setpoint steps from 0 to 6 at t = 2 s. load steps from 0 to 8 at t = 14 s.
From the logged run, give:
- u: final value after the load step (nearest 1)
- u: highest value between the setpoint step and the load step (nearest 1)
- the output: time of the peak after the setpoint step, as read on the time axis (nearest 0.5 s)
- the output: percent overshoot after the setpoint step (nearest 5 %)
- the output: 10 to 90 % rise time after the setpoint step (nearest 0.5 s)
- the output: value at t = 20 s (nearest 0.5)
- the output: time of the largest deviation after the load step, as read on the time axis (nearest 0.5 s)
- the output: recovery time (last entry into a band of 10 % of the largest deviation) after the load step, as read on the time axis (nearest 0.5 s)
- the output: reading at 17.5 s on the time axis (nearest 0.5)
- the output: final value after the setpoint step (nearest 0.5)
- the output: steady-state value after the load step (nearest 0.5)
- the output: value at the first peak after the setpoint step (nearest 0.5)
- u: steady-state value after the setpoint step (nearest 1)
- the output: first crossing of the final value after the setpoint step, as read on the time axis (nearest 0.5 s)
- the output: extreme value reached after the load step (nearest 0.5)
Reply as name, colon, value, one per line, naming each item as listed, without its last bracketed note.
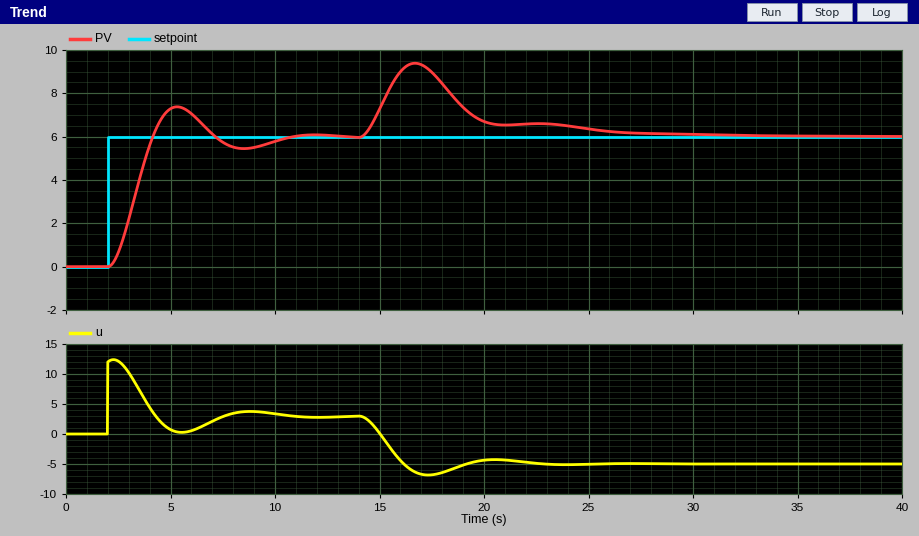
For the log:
u: final value after the load step: -5
u: highest value between the setpoint step and the load step: 12
the output: time of the peak after the setpoint step, as read on the time axis: 5.5 s
the output: percent overshoot after the setpoint step: 25 %
the output: 10 to 90 % rise time after the setpoint step: 1.5 s
the output: value at t = 20 s: 6.5
the output: time of the largest deviation after the load step, as read on the time axis: 16.5 s
the output: recovery time (last entry into a band of 10 % of the largest deviation) after the load step, as read on the time axis: 25.0 s
the output: reading at 17.5 s on the time axis: 9.0
the output: final value after the setpoint step: 6.0
the output: steady-state value after the load step: 6.0
the output: value at the first peak after the setpoint step: 7.5
u: steady-state value after the setpoint step: 3
the output: first crossing of the final value after the setpoint step, as read on the time axis: 4.0 s
the output: extreme value reached after the load step: 9.5
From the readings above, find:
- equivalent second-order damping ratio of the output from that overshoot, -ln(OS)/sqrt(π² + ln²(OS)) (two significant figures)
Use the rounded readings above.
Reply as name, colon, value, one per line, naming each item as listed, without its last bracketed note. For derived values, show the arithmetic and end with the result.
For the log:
equivalent second-order damping ratio of the output from that overshoot, -ln(OS)/sqrt(π² + ln²(OS)): ln(0.25) = -1.386; 1.386 / sqrt(9.870 + 1.922) = 0.40
